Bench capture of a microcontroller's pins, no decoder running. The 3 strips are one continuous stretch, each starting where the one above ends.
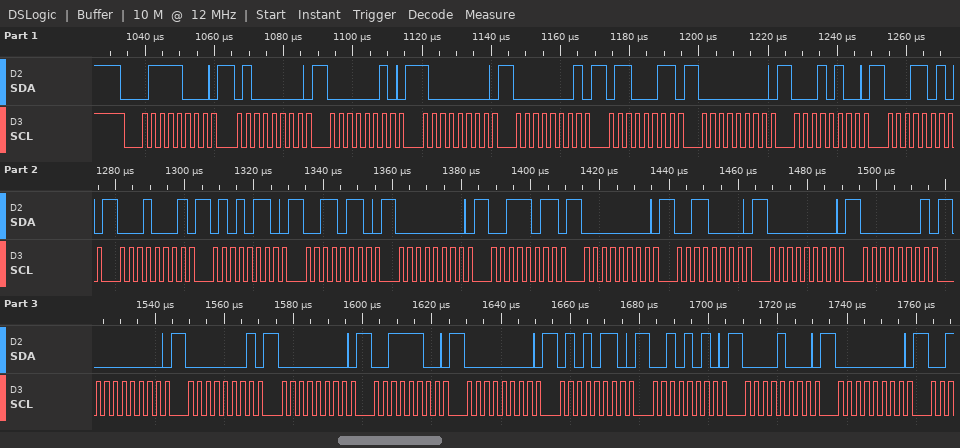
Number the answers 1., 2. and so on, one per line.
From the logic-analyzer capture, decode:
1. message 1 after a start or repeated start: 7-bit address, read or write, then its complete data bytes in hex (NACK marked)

1. 0x3C write: 40 02 80 01 63 00 14 1A 11 56 36 00 3B 00 30 00 01 00 01 00 3C 00 56 2A 08 00
